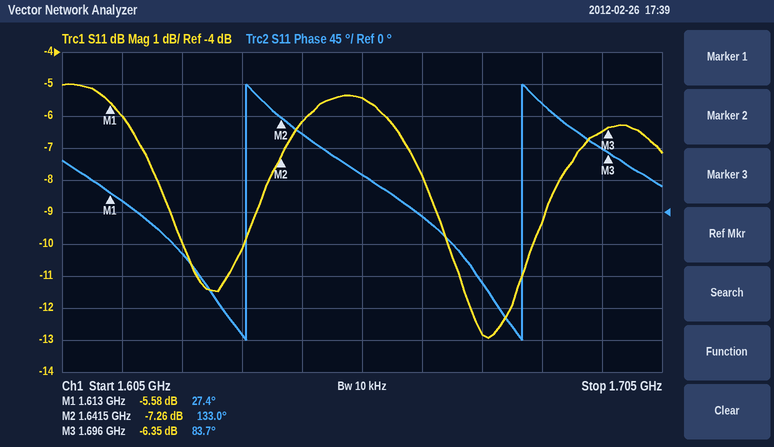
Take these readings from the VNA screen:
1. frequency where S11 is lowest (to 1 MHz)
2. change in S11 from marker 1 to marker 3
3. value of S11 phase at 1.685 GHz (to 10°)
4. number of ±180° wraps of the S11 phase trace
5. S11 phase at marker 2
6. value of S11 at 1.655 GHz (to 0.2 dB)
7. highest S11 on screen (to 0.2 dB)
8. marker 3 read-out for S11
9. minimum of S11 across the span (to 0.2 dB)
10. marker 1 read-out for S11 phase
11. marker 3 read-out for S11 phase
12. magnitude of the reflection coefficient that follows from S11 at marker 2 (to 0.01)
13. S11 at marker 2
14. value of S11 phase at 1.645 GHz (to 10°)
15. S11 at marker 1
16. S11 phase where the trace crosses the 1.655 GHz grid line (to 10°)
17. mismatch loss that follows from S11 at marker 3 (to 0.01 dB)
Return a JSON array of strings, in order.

["1.676 GHz", "-0.77 dB", "150°", "2", "133.0°", "-5.4 dB", "-5.0 dB", "-6.35 dB", "-13.0 dB", "27.4°", "83.7°", "0.43", "-7.26 dB", "110°", "-5.58 dB", "50°", "1.14 dB"]
